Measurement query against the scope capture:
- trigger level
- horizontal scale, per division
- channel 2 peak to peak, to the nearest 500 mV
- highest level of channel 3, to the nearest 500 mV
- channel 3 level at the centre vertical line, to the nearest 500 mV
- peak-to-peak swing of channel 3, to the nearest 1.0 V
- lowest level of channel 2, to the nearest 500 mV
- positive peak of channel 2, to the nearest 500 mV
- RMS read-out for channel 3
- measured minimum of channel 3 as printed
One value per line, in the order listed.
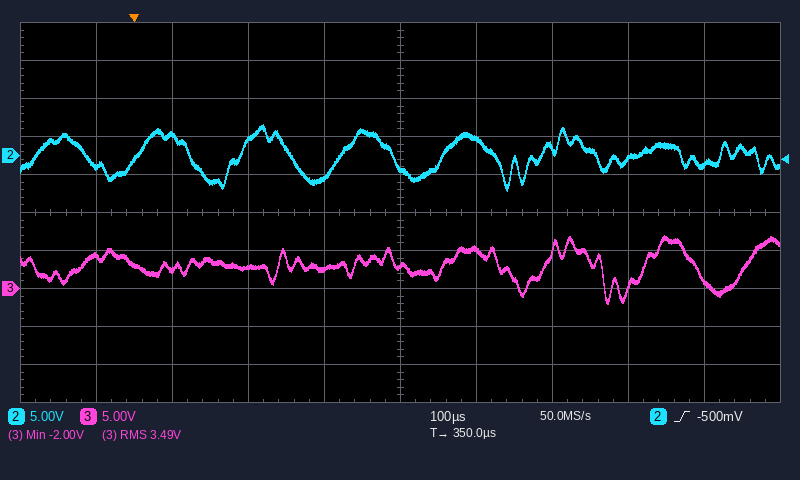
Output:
-500 mV
100 µs
8.5 V
7.0 V
3.0 V
9.0 V
-4.5 V
4.0 V
3.49 V
-2.00 V
